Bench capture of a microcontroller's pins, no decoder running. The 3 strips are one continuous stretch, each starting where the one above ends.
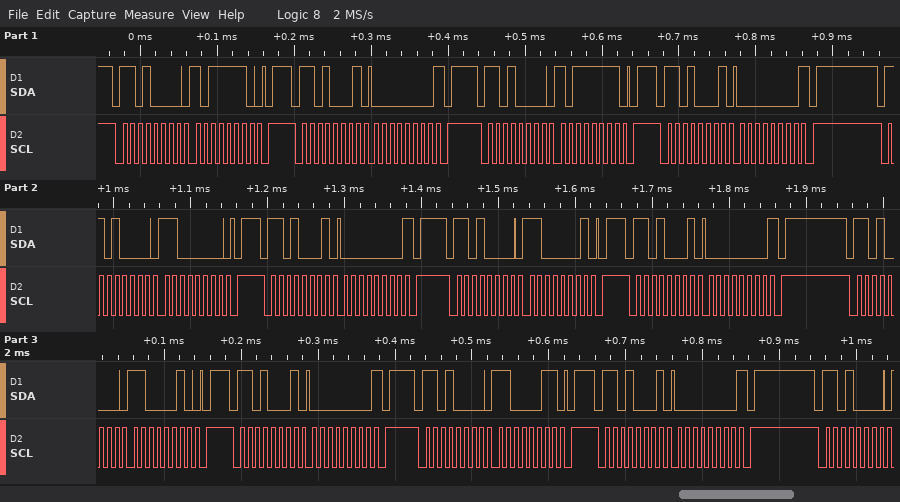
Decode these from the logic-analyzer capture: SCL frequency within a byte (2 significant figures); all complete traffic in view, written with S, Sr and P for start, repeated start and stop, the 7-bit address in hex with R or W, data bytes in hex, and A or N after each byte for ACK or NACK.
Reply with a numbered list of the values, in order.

1. 100 kHz
2. S 68W A BE A P S 68R A 00 N P S 68W A BF A P S 68R A 00 N P S 68W A C0 A P S 68R A 00 N P S 68W A C1 A P S 68R A 00 N P S 68W A C2 A P S 68R A 00 N P S 68W A C3 A P S 68R A 00 N P S 68W A
